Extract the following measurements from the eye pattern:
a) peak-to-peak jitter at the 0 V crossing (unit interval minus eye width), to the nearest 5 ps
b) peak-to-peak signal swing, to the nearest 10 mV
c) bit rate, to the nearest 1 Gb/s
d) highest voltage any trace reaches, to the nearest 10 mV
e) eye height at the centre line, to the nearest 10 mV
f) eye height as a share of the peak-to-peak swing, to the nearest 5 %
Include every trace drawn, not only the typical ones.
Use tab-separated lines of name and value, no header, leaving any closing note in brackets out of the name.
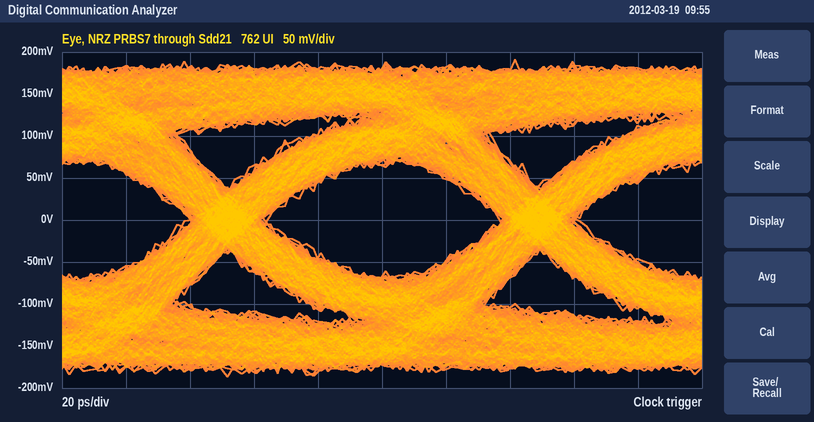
peak-to-peak jitter at the 0 V crossing (unit interval minus eye width), to the nearest 5 ps	25 ps
peak-to-peak signal swing, to the nearest 10 mV	380 mV
bit rate, to the nearest 1 Gb/s	10 Gb/s
highest voltage any trace reaches, to the nearest 10 mV	190 mV
eye height at the centre line, to the nearest 10 mV	130 mV
eye height as a share of the peak-to-peak swing, to the nearest 5 %	35 %
